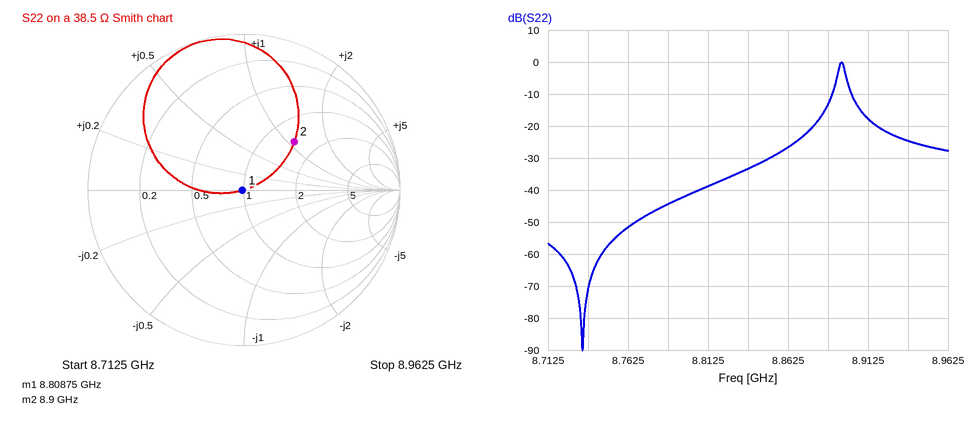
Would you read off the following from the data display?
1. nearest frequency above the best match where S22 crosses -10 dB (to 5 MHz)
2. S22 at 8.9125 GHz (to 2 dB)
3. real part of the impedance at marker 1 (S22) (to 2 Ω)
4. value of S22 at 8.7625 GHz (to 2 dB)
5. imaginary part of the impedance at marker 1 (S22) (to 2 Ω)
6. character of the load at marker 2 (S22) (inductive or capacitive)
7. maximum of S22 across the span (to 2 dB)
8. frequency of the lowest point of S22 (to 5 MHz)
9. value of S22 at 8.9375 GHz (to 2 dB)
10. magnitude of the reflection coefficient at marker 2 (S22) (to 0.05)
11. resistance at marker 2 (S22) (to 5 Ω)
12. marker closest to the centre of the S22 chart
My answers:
8.890 GHz
-18 dB
38 Ω
-52 dB
0 Ω
inductive
0 dB
8.735 GHz
-24 dB
0.45
55 Ω
marker 1
